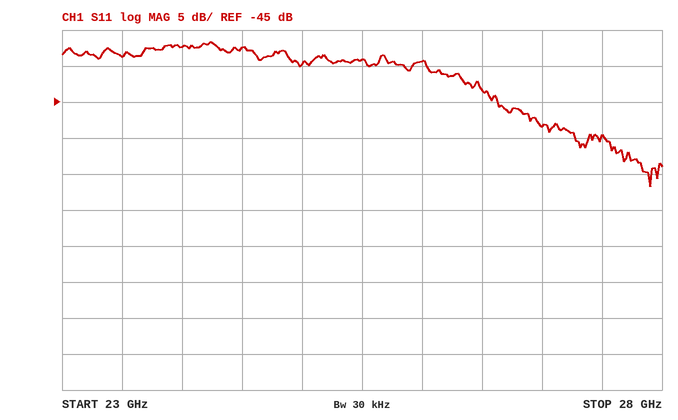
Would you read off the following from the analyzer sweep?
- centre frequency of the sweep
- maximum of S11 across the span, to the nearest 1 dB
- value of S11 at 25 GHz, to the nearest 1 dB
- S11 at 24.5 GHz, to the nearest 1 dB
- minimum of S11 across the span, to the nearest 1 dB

25.5 GHz
-37 dB
-40 dB
-37 dB
-57 dB
